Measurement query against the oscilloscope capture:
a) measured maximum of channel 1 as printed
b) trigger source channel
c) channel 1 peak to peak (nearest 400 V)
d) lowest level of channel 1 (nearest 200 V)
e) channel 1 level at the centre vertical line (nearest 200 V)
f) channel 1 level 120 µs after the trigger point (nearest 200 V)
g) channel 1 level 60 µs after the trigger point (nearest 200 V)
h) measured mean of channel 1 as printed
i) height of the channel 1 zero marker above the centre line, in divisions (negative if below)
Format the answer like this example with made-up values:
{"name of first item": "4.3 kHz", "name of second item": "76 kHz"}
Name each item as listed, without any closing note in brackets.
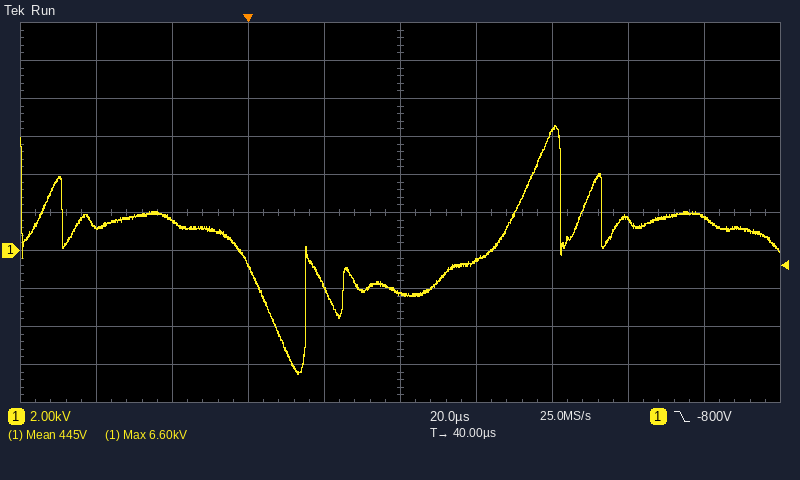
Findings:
{"measured maximum of channel 1 as printed": "6.60 kV", "trigger source channel": "channel 1", "channel 1 peak to peak": "13.2 kV", "lowest level of channel 1": "-6.6 kV", "channel 1 level at the centre vertical line": "-2.2 kV", "channel 1 level 120 µs after the trigger point": "1.8 kV", "channel 1 level 60 µs after the trigger point": "-600 V", "measured mean of channel 1 as printed": "445 V", "height of the channel 1 zero marker above the centre line, in divisions": "-1.0 div"}
